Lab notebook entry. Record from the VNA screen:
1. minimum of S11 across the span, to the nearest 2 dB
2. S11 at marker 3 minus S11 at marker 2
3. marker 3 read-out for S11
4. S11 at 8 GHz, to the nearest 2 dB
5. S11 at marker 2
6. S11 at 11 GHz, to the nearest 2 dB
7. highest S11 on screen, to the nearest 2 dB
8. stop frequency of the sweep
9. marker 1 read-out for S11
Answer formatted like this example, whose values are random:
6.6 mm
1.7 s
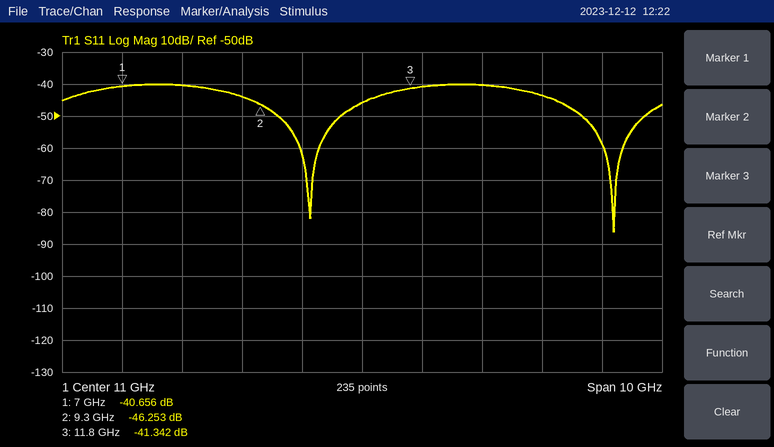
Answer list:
-86 dB
4.911 dB
-41.342 dB
-40 dB
-46.253 dB
-46 dB
-40 dB
16 GHz
-40.656 dB
